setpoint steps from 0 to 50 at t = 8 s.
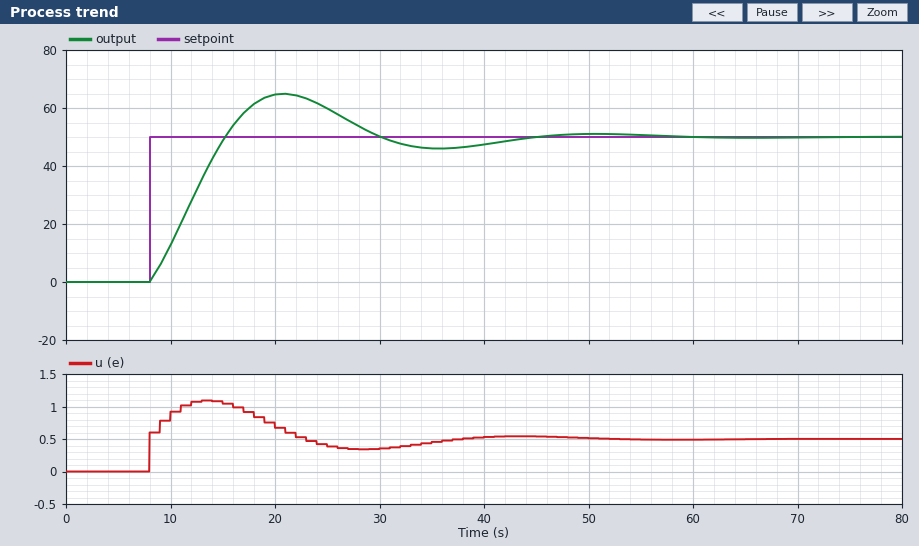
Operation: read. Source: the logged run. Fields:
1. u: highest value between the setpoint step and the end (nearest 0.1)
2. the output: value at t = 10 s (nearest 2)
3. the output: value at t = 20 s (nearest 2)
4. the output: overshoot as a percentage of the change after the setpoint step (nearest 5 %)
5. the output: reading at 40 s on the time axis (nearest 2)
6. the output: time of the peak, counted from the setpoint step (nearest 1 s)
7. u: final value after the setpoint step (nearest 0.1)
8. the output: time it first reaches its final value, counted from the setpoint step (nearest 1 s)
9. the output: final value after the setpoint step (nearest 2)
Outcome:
1.1
12
64
30 %
48
13 s
0.5
7 s
50
